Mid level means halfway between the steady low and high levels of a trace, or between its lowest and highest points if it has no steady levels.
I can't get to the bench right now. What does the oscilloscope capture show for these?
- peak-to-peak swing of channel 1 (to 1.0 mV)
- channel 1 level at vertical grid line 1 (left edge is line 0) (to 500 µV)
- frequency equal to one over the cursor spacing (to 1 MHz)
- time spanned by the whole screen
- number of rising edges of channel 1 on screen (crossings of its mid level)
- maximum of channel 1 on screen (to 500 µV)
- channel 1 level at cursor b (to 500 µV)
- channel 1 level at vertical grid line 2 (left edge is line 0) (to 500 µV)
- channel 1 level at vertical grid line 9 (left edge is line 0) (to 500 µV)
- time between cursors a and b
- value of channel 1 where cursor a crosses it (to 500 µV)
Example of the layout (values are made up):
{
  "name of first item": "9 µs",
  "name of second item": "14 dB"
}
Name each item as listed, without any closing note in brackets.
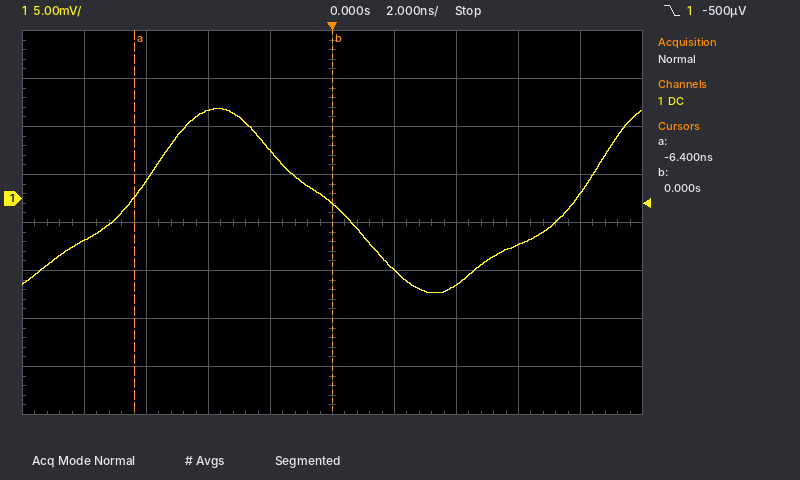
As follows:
{
  "peak-to-peak swing of channel 1": "19.0 mV",
  "channel 1 level at vertical grid line 1 (left edge is line 0)": "-4.5 mV",
  "frequency equal to one over the cursor spacing": "156 MHz",
  "time spanned by the whole screen": "20 ns",
  "number of rising edges of channel 1 on screen": "2",
  "maximum of channel 1 on screen": "9.5 mV",
  "channel 1 level at cursor b": "-500 µV",
  "channel 1 level at vertical grid line 2 (left edge is line 0)": "2.0 mV",
  "channel 1 level at vertical grid line 9 (left edge is line 0)": "500 µV",
  "time between cursors a and b": "6.4 ns",
  "value of channel 1 where cursor a crosses it": "0.0 mV"
}
